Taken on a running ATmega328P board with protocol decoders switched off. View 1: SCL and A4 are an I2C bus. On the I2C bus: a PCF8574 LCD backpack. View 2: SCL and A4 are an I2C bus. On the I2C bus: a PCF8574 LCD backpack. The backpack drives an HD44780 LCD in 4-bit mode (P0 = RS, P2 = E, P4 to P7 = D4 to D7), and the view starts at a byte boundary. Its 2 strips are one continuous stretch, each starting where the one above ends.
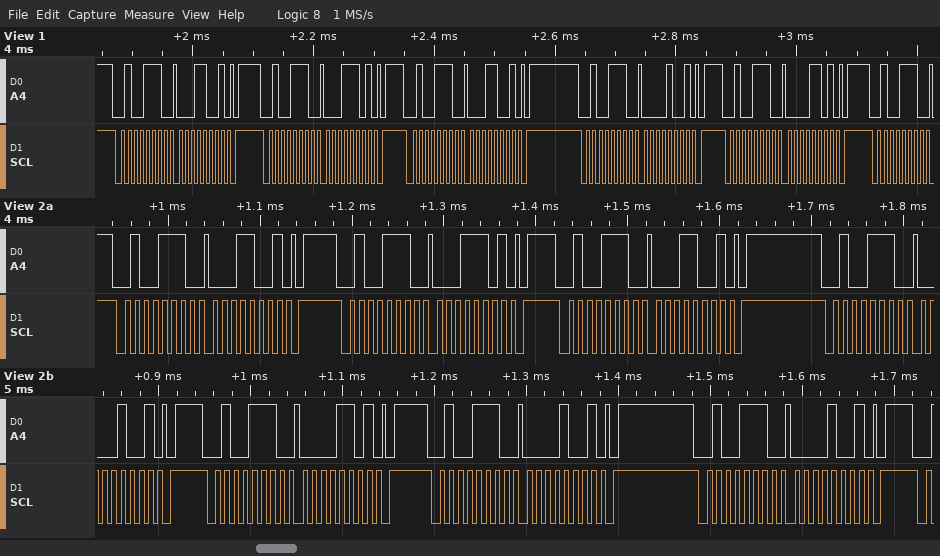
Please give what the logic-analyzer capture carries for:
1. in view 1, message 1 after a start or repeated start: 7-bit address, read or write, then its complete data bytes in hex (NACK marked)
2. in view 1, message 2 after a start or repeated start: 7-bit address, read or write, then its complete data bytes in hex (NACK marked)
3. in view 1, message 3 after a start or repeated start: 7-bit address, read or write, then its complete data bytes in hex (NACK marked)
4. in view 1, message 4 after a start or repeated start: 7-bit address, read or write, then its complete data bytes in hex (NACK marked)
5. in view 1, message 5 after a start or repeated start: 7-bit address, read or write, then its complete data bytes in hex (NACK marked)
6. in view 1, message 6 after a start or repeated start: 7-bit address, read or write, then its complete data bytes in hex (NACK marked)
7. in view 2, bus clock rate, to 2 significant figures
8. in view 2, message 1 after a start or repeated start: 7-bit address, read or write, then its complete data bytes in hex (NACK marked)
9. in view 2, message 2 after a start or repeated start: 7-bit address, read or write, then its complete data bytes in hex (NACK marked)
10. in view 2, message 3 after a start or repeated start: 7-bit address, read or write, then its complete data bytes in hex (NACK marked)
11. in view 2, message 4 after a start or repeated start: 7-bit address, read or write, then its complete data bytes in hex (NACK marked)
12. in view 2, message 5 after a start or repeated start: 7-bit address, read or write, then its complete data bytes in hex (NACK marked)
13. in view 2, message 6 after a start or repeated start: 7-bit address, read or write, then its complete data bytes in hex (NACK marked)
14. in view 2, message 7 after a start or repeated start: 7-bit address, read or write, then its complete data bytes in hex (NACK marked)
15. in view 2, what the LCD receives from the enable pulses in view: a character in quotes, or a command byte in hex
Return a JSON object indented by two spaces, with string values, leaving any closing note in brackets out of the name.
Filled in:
{
  "in view 1, message 1 after a start or repeated start: 7-bit address, read or write, then its complete data bytes in hex": "0x27 write: 19",
  "in view 1, message 2 after a start or repeated start: 7-bit address, read or write, then its complete data bytes in hex": "0x27 write: 1D",
  "in view 1, message 3 after a start or repeated start: 7-bit address, read or write, then its complete data bytes in hex": "0x27 write: 19",
  "in view 1, message 4 after a start or repeated start: 7-bit address, read or write, then its complete data bytes in hex": "0x27 write: 09",
  "in view 1, message 5 after a start or repeated start: 7-bit address, read or write, then its complete data bytes in hex": "0x27 write: 0D",
  "in view 1, message 6 after a start or repeated start: 7-bit address, read or write, then its complete data bytes in hex": "0x27 write",
  "in view 2, bus clock rate, to 2 significant figures": "100 kHz",
  "in view 2, message 1 after a start or repeated start: 7-bit address, read or write, then its complete data bytes in hex": "0x27 write: 19",
  "in view 2, message 2 after a start or repeated start: 7-bit address, read or write, then its complete data bytes in hex": "0x27 write: 1D",
  "in view 2, message 3 after a start or repeated start: 7-bit address, read or write, then its complete data bytes in hex": "0x27 write: 19",
  "in view 2, message 4 after a start or repeated start: 7-bit address, read or write, then its complete data bytes in hex": "0x27 write: 09",
  "in view 2, message 5 after a start or repeated start: 7-bit address, read or write, then its complete data bytes in hex": "0x27 write: 0D",
  "in view 2, message 6 after a start or repeated start: 7-bit address, read or write, then its complete data bytes in hex": "0x27 write: 09",
  "in view 2, message 7 after a start or repeated start: 7-bit address, read or write, then its complete data bytes in hex": "0x27 write: 09",
  "in view 2, what the LCD receives from the enable pulses in view: a character in quotes, or a command byte in hex": "data 0x10"
}
